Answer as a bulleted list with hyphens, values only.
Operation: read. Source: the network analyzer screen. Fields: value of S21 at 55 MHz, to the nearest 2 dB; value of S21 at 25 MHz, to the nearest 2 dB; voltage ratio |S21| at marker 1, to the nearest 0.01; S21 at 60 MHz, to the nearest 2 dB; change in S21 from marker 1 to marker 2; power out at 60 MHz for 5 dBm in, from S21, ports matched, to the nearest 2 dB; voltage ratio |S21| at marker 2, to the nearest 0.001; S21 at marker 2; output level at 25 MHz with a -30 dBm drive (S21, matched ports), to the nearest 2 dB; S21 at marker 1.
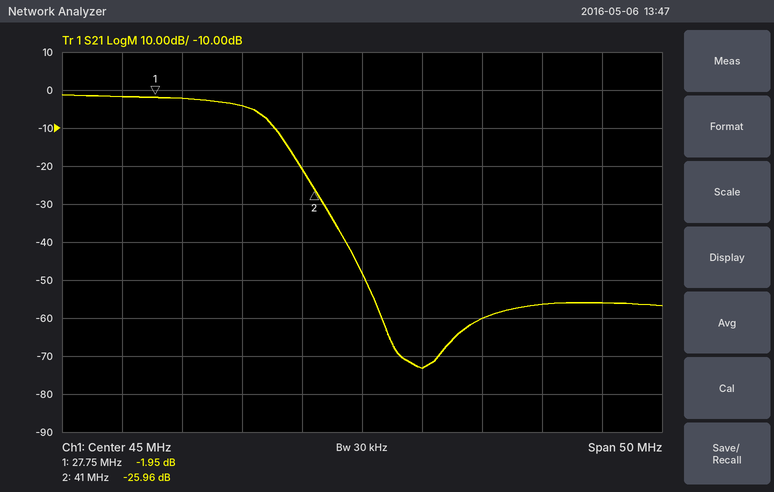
- -60 dB
- -2 dB
- 0.80
- -56 dB
- -24.01 dB
- -52 dBm
- 0.050
- -25.96 dB
- -32 dBm
- -1.95 dB
